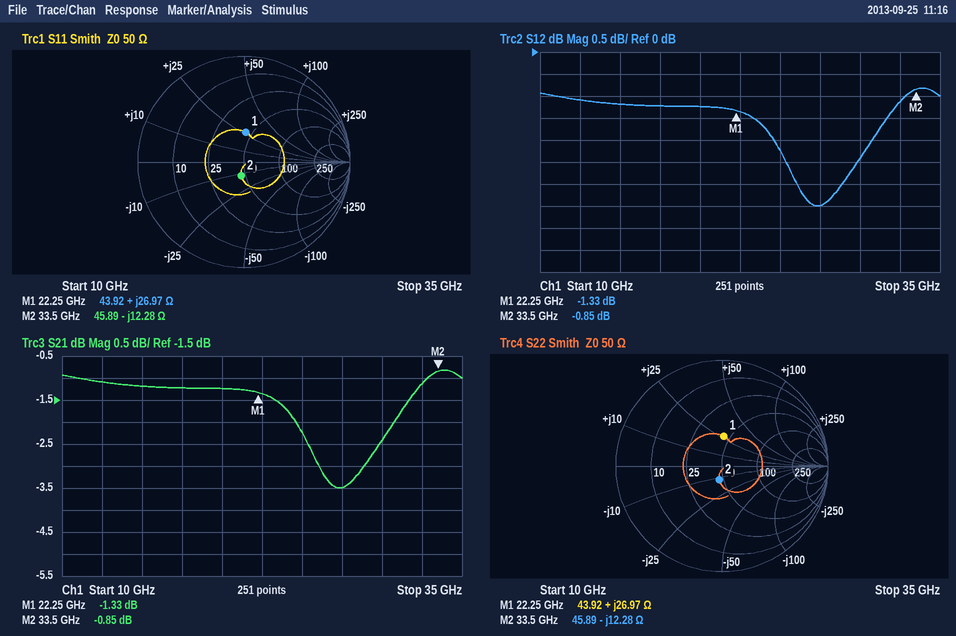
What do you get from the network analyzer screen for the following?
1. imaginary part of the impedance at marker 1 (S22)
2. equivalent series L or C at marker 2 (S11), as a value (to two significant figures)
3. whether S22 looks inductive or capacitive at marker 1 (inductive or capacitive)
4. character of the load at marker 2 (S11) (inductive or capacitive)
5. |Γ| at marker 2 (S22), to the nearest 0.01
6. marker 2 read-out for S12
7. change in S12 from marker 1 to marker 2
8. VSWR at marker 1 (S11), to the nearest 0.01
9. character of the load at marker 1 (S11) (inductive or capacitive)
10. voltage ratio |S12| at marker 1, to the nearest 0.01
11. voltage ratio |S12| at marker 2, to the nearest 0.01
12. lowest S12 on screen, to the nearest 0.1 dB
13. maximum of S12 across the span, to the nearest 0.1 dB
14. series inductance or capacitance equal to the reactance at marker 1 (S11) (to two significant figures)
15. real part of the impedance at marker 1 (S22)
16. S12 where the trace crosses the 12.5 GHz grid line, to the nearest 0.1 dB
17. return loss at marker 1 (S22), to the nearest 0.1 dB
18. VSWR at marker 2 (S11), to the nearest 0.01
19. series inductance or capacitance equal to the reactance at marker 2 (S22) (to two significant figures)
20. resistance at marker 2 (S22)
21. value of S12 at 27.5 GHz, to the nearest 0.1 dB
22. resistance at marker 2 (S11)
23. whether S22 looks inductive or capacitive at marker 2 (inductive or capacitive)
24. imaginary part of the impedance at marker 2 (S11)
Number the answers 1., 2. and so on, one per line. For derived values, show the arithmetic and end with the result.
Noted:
1. +26.97 Ω
2. C = 1/(2π × 33.5 GHz × 12.28 Ω) ≈ 387 fF, so 390 fF to two significant figures
3. inductive
4. capacitive
5. 0.13
6. -0.85 dB
7. -0.85 − (-1.33) = 0.48 dB
8. 1.79
9. inductive
10. 10^(-1.33/20) ≈ 0.86
11. 10^(-0.85/20) ≈ 0.91
12. -3.5 dB
13. -0.8 dB
14. L = 26.97 Ω/(2π × 22.25 GHz) ≈ 193 pH, so 190 pH to two significant figures
15. 43.92 Ω
16. -1.1 dB
17. 11.0 dB
18. 1.31
19. C = 1/(2π × 33.5 GHz × 12.28 Ω) ≈ 387 fF, so 390 fF to two significant figures
20. 45.89 Ω
21. -3.5 dB
22. 45.89 Ω
23. capacitive
24. -12.28 Ω
